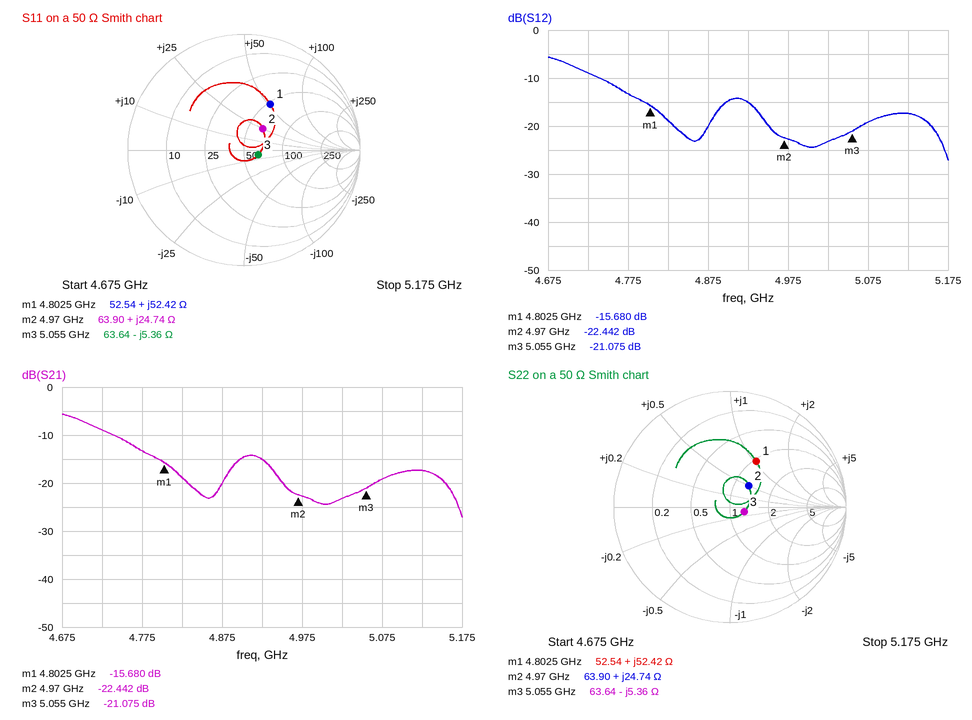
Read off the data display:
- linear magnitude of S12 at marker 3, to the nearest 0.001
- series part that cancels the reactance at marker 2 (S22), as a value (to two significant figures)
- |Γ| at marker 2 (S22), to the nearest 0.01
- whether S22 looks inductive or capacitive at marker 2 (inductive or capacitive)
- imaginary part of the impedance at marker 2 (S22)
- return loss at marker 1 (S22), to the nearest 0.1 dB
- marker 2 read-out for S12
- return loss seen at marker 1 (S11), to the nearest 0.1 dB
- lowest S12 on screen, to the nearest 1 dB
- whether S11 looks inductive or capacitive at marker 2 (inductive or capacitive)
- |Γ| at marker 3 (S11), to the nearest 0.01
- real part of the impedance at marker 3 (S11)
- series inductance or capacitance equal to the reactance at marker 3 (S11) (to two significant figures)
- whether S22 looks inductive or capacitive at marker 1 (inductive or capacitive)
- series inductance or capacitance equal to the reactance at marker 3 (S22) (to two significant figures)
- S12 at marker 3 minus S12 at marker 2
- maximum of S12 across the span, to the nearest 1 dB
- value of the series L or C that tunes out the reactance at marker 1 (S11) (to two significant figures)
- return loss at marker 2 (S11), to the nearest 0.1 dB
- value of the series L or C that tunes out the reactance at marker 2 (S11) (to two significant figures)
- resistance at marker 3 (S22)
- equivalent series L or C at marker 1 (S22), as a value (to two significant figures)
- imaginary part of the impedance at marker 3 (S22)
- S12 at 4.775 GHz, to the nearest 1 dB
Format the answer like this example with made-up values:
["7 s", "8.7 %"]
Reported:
["0.088", "1.3 pF", "0.24", "inductive", "+24.74 Ω", "6.8 dB", "-22.442 dB", "6.8 dB", "-27 dB", "inductive", "0.13", "63.64 Ω", "5.9 pF", "inductive", "5.9 pF", "1.367 dB", "-6 dB", "630 fF", "12.3 dB", "1.3 pF", "63.64 Ω", "1.7 nH", "-5.36 Ω", "-13 dB"]
